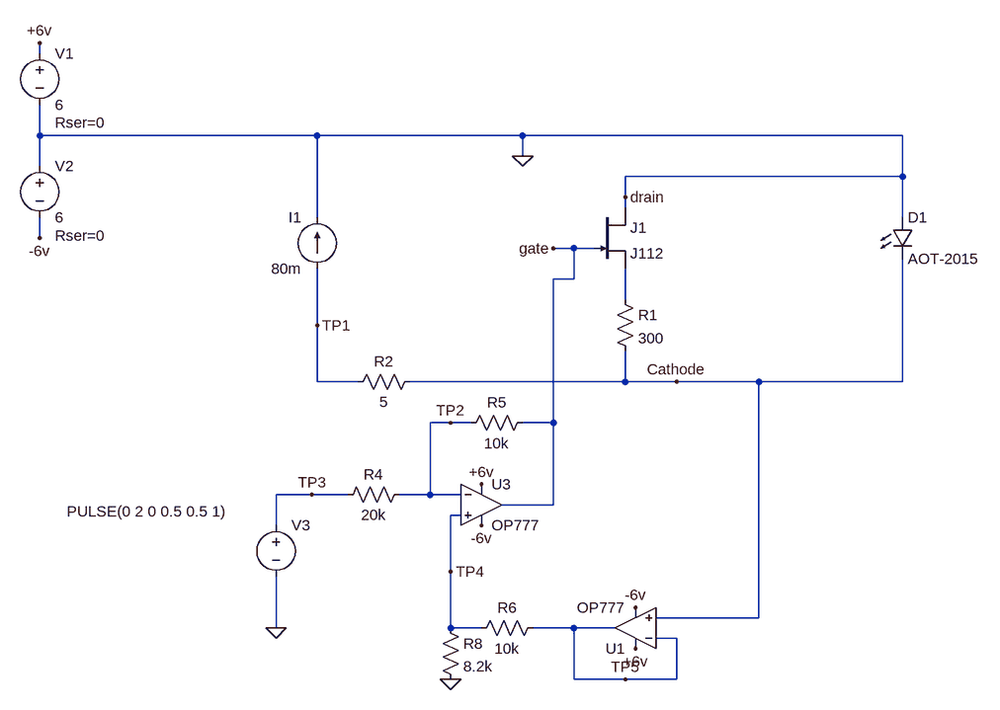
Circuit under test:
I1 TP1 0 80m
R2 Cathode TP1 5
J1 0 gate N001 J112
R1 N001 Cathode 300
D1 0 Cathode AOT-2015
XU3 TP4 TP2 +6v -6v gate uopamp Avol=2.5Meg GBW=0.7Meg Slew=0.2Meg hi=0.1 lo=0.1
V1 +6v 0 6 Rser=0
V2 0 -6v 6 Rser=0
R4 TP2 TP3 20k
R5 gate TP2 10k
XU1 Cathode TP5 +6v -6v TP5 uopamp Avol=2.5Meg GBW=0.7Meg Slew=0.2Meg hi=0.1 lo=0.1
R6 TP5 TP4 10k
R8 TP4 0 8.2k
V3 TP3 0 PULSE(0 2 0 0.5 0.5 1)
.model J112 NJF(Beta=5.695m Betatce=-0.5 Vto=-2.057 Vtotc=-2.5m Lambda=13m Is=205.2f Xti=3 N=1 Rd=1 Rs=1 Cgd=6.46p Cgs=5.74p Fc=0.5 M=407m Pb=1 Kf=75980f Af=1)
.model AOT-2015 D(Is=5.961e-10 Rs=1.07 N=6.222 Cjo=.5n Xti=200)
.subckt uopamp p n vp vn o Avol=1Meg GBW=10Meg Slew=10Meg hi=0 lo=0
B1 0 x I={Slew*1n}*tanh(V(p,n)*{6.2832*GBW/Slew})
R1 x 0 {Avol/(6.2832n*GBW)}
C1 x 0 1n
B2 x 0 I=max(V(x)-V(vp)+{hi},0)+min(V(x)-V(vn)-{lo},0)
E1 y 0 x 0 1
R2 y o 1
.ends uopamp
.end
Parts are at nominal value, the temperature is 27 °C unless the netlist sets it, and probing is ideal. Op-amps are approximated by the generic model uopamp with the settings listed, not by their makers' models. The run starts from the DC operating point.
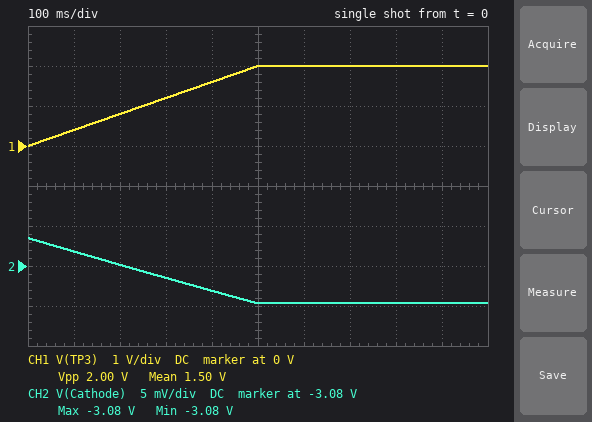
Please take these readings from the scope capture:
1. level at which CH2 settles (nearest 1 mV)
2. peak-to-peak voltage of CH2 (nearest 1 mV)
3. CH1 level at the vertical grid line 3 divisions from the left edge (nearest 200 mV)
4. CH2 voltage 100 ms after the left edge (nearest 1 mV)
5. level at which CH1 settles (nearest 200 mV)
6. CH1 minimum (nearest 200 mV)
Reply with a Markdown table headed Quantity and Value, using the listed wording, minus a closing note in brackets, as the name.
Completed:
| Quantity | Value |
|---|---|
| level at which CH2 settles | -3.085 V |
| peak-to-peak voltage of CH2 | 8 mV |
| CH1 level at the vertical grid line 3 divisions from the left edge | 1.2 V |
| CH2 voltage 100 ms after the left edge | -3.078 V |
| level at which CH1 settles | 2.0 V |
| CH1 minimum | 0 V |
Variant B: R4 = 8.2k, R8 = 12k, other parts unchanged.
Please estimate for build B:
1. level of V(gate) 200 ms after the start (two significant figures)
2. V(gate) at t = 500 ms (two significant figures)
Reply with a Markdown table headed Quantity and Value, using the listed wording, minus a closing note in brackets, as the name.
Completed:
| Quantity | Value |
|---|---|
| level of V(gate) 200 ms after the start | -4.7 V |
| V(gate) at t = 500 ms | -5.9 V |
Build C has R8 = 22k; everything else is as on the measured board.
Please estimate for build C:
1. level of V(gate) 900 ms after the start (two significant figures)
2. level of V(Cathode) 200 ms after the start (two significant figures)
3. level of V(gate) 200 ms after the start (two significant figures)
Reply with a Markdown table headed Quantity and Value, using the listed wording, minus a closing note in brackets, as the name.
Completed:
| Quantity | Value |
|---|---|
| level of V(gate) 900 ms after the start | -4.2 V |
| level of V(Cathode) 200 ms after the start | -3.1 V |
| level of V(gate) 200 ms after the start | -3.6 V |
